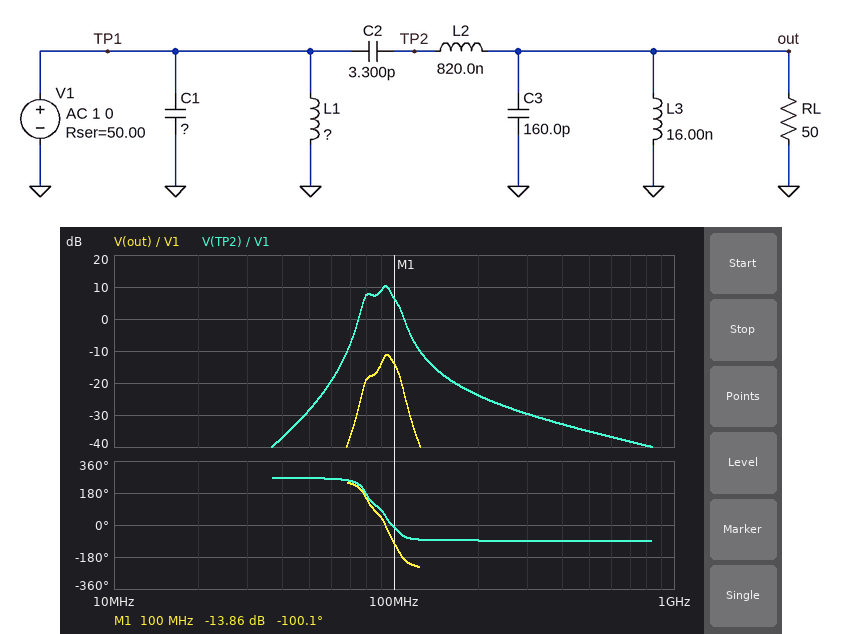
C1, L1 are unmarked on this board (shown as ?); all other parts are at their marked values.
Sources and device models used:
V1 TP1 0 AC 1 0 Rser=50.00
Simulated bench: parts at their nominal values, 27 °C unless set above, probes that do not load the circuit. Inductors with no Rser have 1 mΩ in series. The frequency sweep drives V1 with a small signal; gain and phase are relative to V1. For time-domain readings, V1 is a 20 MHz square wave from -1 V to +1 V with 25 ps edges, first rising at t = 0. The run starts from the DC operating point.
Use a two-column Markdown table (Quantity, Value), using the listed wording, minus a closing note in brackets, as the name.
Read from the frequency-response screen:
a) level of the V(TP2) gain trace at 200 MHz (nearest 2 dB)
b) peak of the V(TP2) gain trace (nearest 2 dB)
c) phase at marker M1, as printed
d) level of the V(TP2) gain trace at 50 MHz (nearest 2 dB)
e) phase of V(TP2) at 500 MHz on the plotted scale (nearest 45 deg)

| Quantity | Value |
|---|---|
| level of the V(TP2) gain trace at 200 MHz | -24 dB |
| peak of the V(TP2) gain trace | 10 dB |
| phase at marker M1, as printed | -100.1 deg |
| level of the V(TP2) gain trace at 50 MHz | -28 dB |
| phase of V(TP2) at 500 MHz on the plotted scale | -90 deg |
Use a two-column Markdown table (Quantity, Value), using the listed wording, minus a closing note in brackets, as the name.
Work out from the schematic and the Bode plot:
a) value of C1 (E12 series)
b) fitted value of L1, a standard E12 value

| Quantity | Value |
|---|---|
| value of C1 | 390 pF |
| fitted value of L1, a standard E12 value | 10 nH |
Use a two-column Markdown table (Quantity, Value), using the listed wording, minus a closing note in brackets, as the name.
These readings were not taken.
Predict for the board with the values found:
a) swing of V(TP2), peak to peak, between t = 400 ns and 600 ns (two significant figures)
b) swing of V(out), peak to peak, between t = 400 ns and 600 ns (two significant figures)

| Quantity | Value |
|---|---|
| swing of V(TP2), peak to peak, between t = 400 ns and 600 ns | 1.1 V |
| swing of V(out), peak to peak, between t = 400 ns and 600 ns | 100 mV |
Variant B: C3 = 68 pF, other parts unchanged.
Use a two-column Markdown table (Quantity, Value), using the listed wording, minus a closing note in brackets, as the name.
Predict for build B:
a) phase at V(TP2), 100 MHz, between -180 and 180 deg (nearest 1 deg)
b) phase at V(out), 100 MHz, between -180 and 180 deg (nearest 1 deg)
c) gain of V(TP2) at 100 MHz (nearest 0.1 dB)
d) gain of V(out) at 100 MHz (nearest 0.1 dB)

| Quantity | Value |
|---|---|
| phase at V(TP2), 100 MHz, between -180 and 180 deg | -65 deg |
| phase at V(out), 100 MHz, between -180 and 180 deg | -84 deg |
| gain of V(TP2) at 100 MHz | 9.9 dB |
| gain of V(out) at 100 MHz | -20.2 dB |
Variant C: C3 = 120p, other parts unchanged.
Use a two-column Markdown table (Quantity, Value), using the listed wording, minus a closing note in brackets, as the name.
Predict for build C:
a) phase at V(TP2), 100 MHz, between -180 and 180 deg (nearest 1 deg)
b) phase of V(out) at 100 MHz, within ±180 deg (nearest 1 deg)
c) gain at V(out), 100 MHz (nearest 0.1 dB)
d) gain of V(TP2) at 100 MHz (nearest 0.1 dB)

| Quantity | Value |
|---|---|
| phase at V(TP2), 100 MHz, between -180 and 180 deg | -53 deg |
| phase of V(out) at 100 MHz, within ±180 deg | -90 deg |
| gain at V(out), 100 MHz | -17.1 dB |
| gain of V(TP2) at 100 MHz | 7.5 dB |
